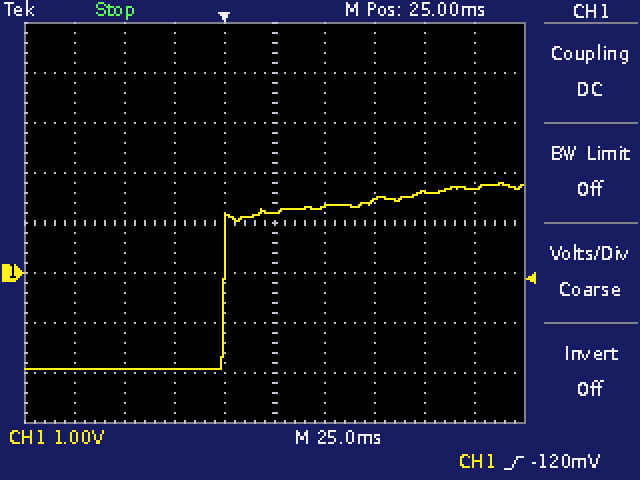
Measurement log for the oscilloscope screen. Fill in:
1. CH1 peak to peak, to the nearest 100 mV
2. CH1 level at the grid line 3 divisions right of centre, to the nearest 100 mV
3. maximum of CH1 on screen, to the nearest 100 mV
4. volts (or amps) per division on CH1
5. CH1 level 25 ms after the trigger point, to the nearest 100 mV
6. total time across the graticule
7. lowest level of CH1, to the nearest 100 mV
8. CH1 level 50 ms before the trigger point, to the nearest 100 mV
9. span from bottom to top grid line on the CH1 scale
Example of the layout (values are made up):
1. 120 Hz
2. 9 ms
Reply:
1. 3.7 V
2. 1.6 V
3. 1.8 V
4. 1 V
5. 1.2 V
6. 250 ms
7. -1.9 V
8. -1.9 V
9. 8 V
